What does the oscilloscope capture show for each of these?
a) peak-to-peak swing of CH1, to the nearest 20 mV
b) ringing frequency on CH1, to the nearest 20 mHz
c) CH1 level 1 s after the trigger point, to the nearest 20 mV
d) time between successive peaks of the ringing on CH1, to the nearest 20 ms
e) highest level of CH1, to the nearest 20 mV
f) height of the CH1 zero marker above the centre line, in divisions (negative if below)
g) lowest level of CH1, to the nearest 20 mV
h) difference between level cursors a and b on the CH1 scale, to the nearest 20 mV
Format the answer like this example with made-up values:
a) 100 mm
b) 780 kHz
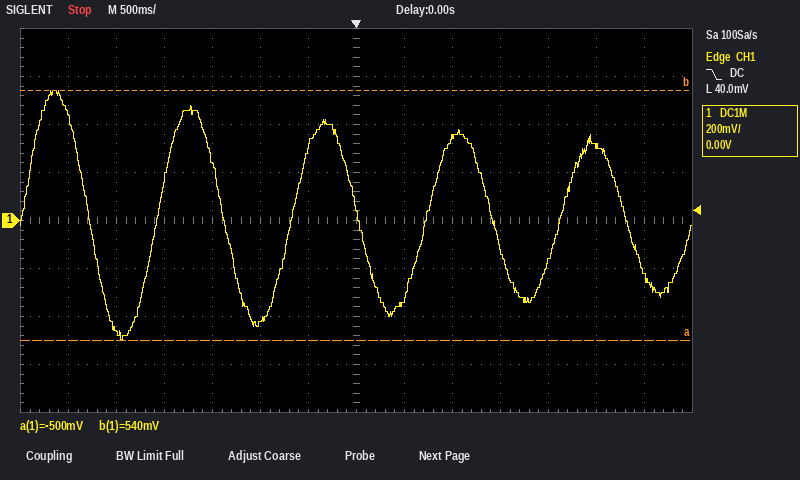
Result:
a) 1.04 V
b) 720 mHz
c) 340 mV
d) 1.40 s
e) 540 mV
f) 0.0 div
g) -500 mV
h) 1.04 V
